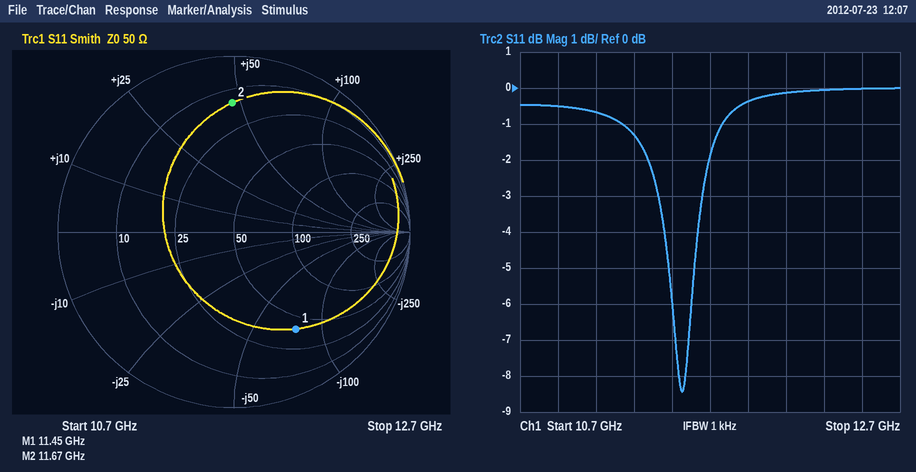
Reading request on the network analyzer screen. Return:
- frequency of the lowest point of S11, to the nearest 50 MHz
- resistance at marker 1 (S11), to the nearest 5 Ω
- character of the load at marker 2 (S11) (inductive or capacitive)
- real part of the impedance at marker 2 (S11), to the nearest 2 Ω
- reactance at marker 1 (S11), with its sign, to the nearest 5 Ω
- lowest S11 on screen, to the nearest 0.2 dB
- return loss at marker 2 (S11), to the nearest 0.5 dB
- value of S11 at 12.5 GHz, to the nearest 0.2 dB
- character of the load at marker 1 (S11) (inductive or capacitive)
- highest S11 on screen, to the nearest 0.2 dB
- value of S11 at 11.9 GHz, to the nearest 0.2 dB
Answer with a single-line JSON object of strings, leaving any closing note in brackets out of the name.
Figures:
{"frequency of the lowest point of S11, to the nearest 50 MHz": "11.55 GHz", "resistance at marker 1 (S11), to the nearest 5 Ω": "40 Ω", "character of the load at marker 2 (S11)": "inductive", "real part of the impedance at marker 2 (S11), to the nearest 2 Ω": "14 Ω", "reactance at marker 1 (S11), with its sign, to the nearest 5 Ω": "-75 Ω", "lowest S11 on screen, to the nearest 0.2 dB": "-8.4 dB", "return loss at marker 2 (S11), to the nearest 0.5 dB": "2.5 dB", "value of S11 at 12.5 GHz, to the nearest 0.2 dB": "0.0 dB", "character of the load at marker 1 (S11)": "capacitive", "highest S11 on screen, to the nearest 0.2 dB": "0.0 dB", "value of S11 at 11.9 GHz, to the nearest 0.2 dB": "-0.4 dB"}
